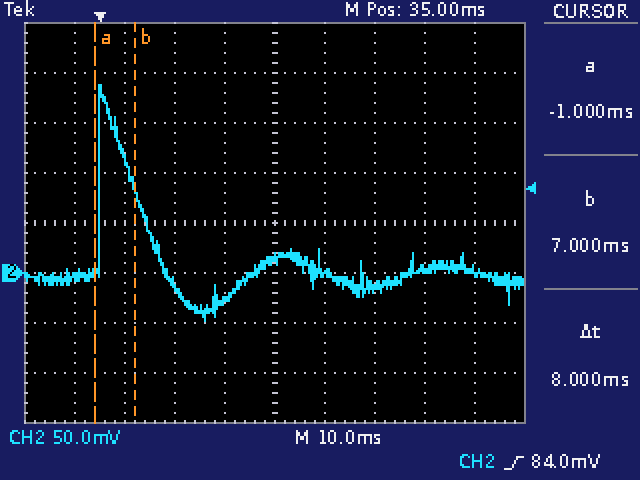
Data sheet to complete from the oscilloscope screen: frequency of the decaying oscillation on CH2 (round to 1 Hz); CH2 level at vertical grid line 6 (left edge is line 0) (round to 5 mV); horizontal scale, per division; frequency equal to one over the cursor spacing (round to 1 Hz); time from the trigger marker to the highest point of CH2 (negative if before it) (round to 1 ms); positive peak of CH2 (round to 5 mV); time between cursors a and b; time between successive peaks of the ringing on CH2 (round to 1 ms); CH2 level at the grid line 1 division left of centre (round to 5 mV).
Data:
28 Hz
0 mV
10 ms
125 Hz
0 ms
190 mV
8 ms
36 ms
-30 mV
